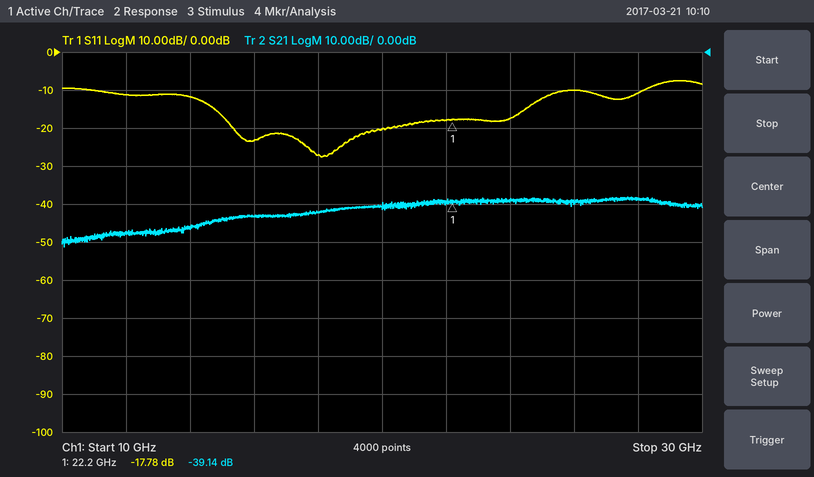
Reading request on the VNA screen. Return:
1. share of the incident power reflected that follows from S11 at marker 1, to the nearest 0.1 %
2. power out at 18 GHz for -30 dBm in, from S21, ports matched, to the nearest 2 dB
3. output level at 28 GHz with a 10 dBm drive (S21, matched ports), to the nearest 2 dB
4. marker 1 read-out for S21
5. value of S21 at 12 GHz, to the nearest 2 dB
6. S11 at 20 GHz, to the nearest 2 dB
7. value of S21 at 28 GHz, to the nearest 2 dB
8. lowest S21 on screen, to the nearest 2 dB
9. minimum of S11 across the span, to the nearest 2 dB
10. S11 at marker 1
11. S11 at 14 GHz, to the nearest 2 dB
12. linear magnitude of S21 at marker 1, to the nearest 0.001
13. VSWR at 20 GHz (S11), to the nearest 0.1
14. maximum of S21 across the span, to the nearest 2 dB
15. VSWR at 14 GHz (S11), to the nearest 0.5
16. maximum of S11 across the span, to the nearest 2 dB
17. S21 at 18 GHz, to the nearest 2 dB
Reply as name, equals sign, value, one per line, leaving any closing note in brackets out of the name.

share of the incident power reflected that follows from S11 at marker 1, to the nearest 0.1 % = 1.7 %
power out at 18 GHz for -30 dBm in, from S21, ports matched, to the nearest 2 dB = -72 dBm
output level at 28 GHz with a 10 dBm drive (S21, matched ports), to the nearest 2 dB = -28 dBm
marker 1 read-out for S21 = -39.14 dB
value of S21 at 12 GHz, to the nearest 2 dB = -48 dB
S11 at 20 GHz, to the nearest 2 dB = -20 dB
value of S21 at 28 GHz, to the nearest 2 dB = -38 dB
lowest S21 on screen, to the nearest 2 dB = -52 dB
minimum of S11 across the span, to the nearest 2 dB = -28 dB
S11 at marker 1 = -17.78 dB
S11 at 14 GHz, to the nearest 2 dB = -12 dB
linear magnitude of S21 at marker 1, to the nearest 0.001 = 0.011
VSWR at 20 GHz (S11), to the nearest 0.1 = 1.2
maximum of S21 across the span, to the nearest 2 dB = -38 dB
VSWR at 14 GHz (S11), to the nearest 0.5 = 1.5
maximum of S11 across the span, to the nearest 2 dB = -8 dB
S21 at 18 GHz, to the nearest 2 dB = -42 dB
